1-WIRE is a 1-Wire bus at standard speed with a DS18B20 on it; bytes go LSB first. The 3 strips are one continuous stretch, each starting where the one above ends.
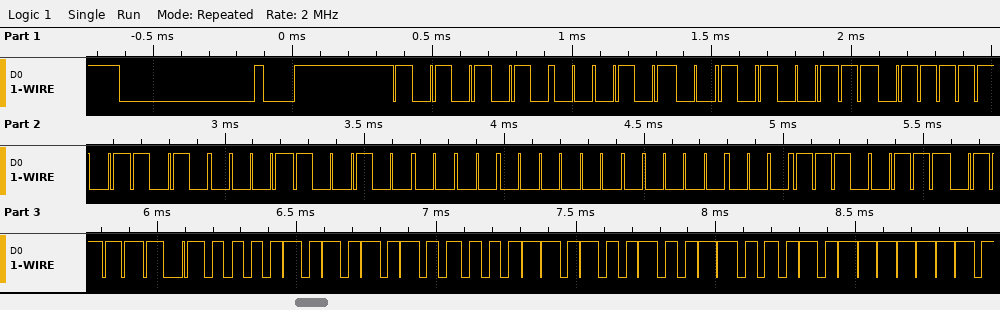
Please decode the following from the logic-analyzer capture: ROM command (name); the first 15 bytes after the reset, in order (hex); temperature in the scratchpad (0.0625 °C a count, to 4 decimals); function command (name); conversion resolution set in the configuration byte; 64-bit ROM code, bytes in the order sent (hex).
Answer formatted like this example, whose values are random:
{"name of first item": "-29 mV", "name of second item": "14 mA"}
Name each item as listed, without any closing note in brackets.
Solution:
{"ROM command": "Match ROM", "the first 15 bytes after the reset, in order": "55 28 E5 BE 85 09 00 00 E7 BE 50 05 4B 46 7F", "temperature in the scratchpad": "85.0000 °C", "function command": "Read Scratchpad", "conversion resolution set in the configuration byte": "12 bits", "64-bit ROM code, bytes in the order sent": "28 E5 BE 85 09 00 00 E7"}
